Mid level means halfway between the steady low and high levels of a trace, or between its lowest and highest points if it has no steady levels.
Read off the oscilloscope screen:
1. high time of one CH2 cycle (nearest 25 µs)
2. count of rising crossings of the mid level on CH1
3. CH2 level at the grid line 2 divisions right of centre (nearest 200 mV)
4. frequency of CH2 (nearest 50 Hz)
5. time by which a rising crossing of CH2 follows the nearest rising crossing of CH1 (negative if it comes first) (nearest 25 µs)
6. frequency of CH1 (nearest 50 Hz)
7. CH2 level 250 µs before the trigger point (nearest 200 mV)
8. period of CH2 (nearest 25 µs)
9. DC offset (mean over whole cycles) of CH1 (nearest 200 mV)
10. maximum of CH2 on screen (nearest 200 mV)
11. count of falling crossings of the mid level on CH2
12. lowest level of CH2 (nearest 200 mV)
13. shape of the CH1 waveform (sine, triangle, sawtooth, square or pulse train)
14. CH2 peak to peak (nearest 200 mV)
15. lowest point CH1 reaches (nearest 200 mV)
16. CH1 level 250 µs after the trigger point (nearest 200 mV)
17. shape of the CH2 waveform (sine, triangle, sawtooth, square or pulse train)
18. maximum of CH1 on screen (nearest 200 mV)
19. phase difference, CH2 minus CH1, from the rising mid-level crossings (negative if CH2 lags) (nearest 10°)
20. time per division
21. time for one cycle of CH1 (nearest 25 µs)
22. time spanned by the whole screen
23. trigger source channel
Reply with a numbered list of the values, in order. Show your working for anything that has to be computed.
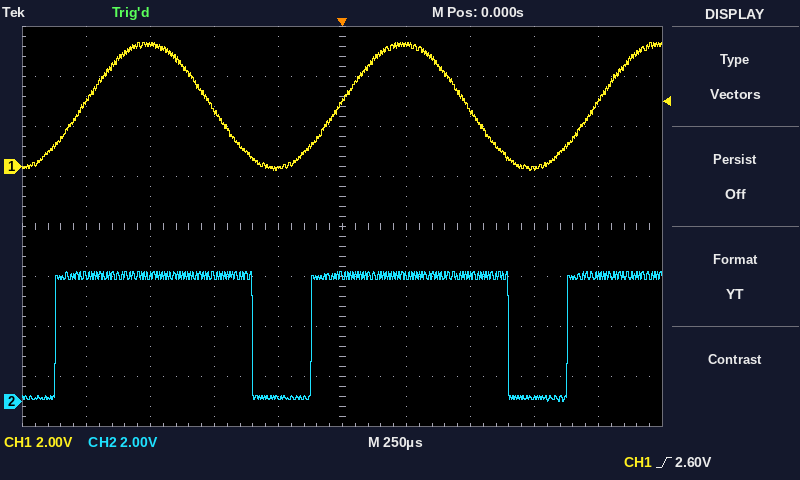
1. 775 µs
2. 3
3. 5.0 V
4. 1 / 1.000 ms ≈ 1.00 kHz
5. -100 µs
6. 1 / 1.000 ms ≈ 1.00 kHz
7. 200 mV
8. 1.000 ms
9. (5.0 V + (-200 mV)) / 2 ≈ 2.4 V
10. 5.2 V
11. 2
12. 0.0 V
13. sine
14. 5.2 V − (0.0 V) = 5.2 V
15. -200 mV
16. 4.8 V
17. pulse train
18. 5.0 V
19. −360° × (-100 µs) / 1.000 ms ≈ +36.0°, so +40° to the nearest 10°
20. 250 µs
21. 1.000 ms
22. 2.5 ms
23. CH1
